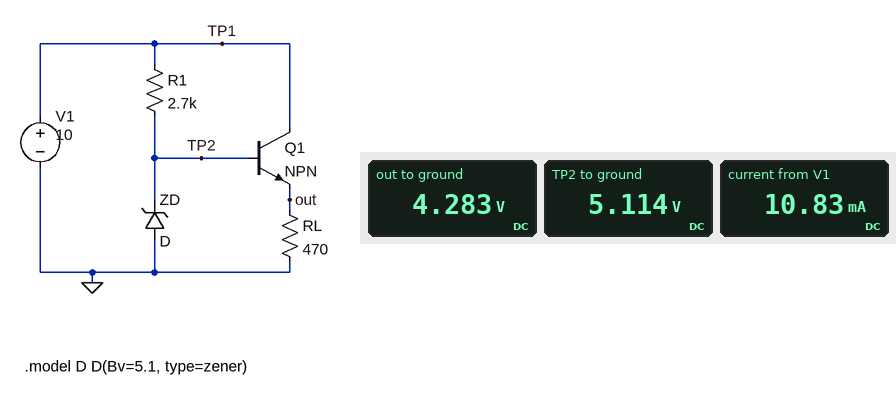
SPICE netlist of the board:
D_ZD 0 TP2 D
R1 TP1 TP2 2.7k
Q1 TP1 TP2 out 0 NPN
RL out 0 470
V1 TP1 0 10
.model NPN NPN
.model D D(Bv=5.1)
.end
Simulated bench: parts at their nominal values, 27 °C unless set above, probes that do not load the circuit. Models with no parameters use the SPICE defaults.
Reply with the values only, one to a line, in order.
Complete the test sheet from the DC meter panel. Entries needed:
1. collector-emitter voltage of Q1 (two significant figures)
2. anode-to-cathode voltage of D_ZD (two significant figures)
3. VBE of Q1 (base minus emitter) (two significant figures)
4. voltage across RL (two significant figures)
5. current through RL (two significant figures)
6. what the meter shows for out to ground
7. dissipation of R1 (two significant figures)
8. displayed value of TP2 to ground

5.7 V
-5.1 V
830 mV
4.3 V
9.1 mA
4.283 V
8.8 mW
5.114 V
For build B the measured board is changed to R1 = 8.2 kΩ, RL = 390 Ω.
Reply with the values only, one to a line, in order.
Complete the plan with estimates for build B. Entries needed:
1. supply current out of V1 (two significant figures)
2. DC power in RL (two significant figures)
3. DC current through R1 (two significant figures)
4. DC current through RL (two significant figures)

11 mA
46 mW
600 µA
11 mA
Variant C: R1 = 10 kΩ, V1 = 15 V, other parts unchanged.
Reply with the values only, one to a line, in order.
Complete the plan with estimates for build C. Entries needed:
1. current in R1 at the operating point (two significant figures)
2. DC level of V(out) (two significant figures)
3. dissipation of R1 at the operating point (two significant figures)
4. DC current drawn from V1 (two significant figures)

990 µA
4.3 V
9.8 mW
10 mA
